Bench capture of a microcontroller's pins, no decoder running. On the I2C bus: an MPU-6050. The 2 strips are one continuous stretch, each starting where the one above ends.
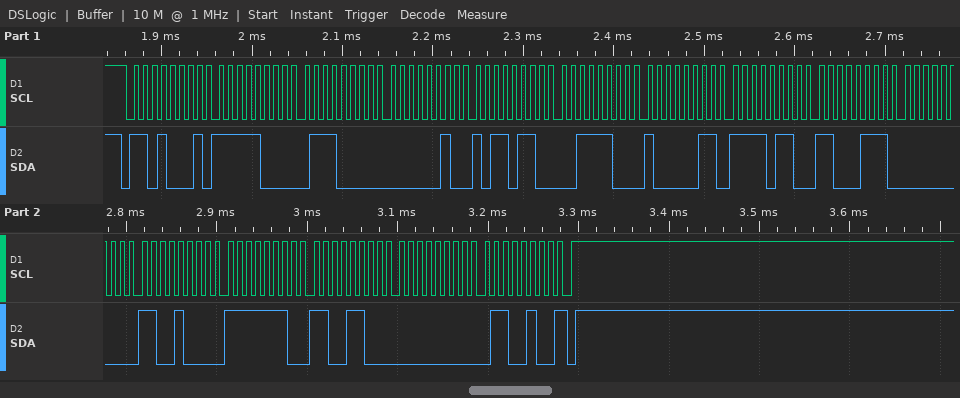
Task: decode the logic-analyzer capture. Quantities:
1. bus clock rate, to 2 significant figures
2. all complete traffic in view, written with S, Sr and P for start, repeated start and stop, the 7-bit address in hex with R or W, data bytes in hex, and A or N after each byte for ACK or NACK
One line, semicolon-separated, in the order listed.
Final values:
100 kHz; S 68R A F8 A 70 A 02 A B6 A 3C A 83 A F6 A C7 A 00 A C8 A FE A CC A 00 A 64 N P
